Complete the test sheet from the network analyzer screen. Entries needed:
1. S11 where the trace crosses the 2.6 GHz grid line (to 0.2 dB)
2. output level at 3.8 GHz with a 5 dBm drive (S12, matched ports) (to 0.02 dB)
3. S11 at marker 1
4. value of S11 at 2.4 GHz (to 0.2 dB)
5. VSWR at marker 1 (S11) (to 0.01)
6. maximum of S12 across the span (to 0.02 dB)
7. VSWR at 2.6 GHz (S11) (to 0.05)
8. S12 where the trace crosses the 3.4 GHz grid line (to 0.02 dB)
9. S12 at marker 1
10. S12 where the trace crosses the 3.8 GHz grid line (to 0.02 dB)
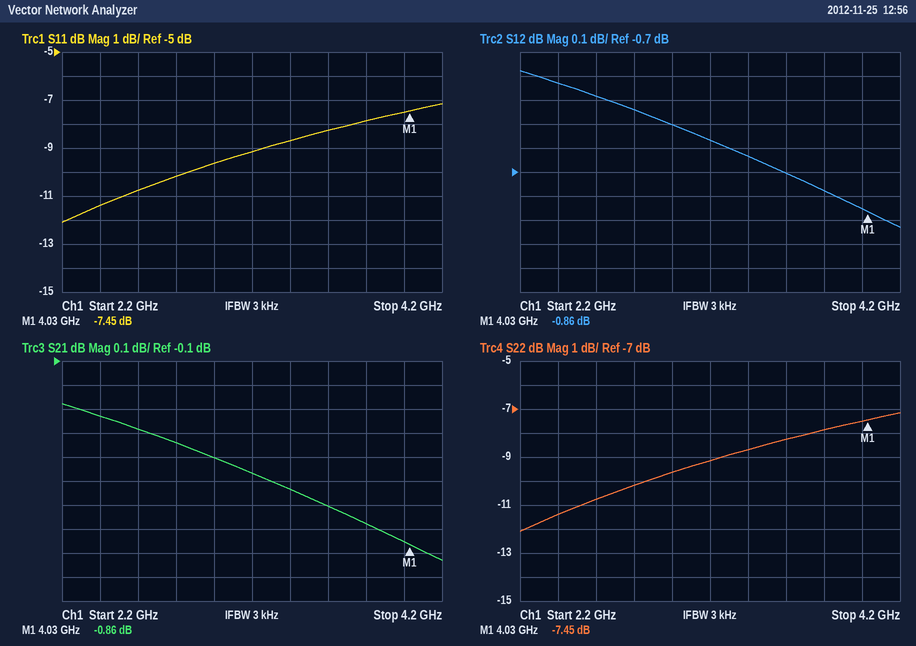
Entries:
-10.8 dB
4.22 dBm
-7.45 dB
-11.4 dB
2.47
-0.28 dB
1.80
-0.64 dB
-0.86 dB
-0.78 dB
